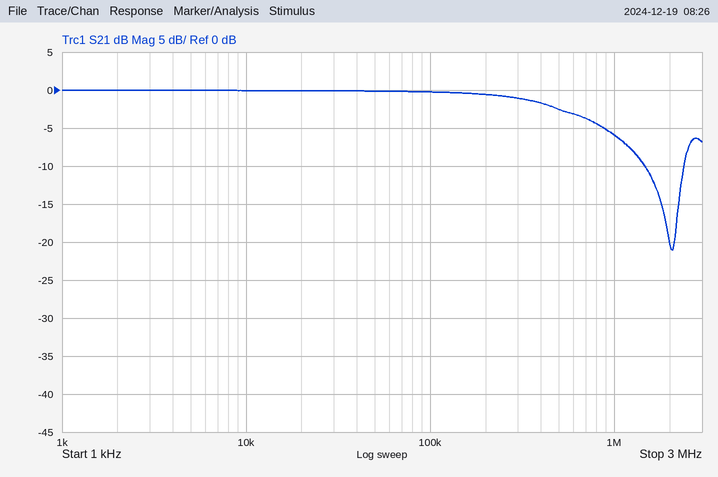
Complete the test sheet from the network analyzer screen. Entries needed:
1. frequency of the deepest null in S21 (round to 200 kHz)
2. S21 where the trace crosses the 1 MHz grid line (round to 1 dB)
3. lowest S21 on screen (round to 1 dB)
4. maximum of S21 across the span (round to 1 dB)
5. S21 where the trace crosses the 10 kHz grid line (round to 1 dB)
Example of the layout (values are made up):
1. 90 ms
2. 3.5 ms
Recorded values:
1. 2.0 MHz
2. -6 dB
3. -21 dB
4. 0 dB
5. 0 dB
